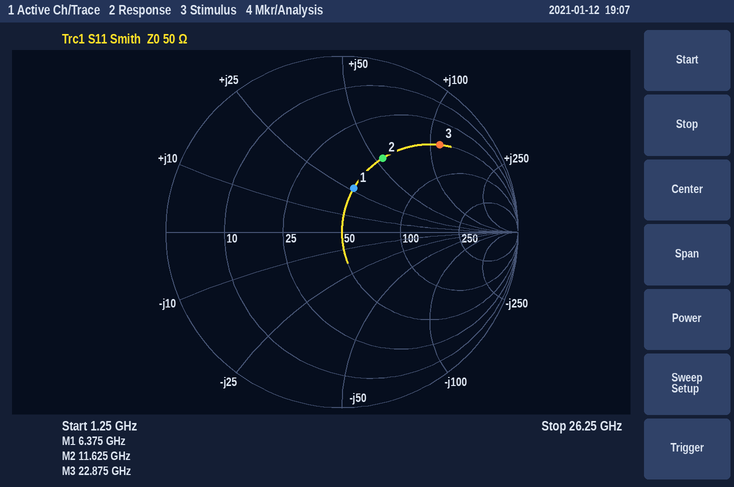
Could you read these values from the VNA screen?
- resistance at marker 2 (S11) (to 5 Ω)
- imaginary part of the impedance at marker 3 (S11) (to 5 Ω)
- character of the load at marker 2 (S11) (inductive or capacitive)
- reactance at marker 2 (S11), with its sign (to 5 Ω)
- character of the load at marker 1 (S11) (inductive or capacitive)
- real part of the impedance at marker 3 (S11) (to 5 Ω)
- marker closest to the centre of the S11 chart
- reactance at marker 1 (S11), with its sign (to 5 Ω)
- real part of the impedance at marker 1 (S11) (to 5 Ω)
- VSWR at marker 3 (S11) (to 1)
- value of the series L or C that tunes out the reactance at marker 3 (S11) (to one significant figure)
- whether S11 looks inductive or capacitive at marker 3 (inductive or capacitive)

50 Ω
+110 Ω
inductive
+55 Ω
inductive
50 Ω
marker 1
+25 Ω
50 Ω
7
60 fF
inductive
